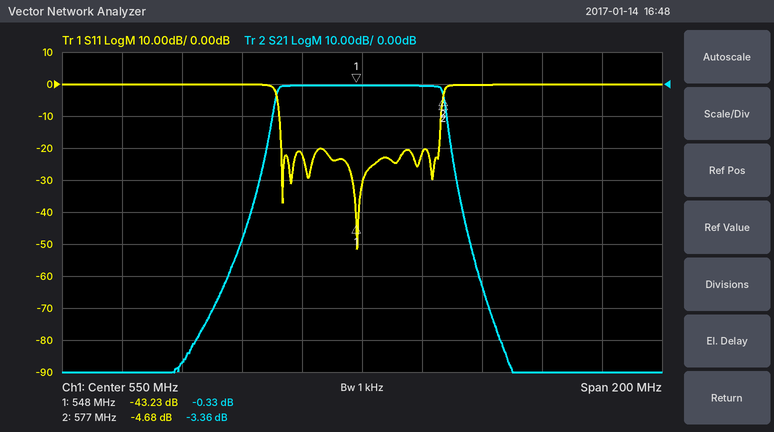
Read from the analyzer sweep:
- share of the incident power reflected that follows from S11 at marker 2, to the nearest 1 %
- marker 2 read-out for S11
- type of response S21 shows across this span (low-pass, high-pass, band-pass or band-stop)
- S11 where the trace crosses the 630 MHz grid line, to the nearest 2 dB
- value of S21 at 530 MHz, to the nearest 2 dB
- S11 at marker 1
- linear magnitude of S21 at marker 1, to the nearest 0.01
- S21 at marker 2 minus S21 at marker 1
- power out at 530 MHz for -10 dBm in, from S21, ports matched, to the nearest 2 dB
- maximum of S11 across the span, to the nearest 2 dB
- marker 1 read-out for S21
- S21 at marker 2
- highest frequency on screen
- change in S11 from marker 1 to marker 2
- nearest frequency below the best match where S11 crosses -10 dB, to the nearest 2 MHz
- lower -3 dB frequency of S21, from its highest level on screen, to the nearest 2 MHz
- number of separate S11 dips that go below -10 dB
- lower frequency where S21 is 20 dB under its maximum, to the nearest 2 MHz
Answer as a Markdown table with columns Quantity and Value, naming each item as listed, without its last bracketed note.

| Quantity | Value |
|---|---|
| share of the incident power reflected that follows from S11 at marker 2, to the nearest 1 % | 34 % |
| marker 2 read-out for S11 | -4.68 dB |
| type of response S21 shows across this span | band-pass |
| S11 where the trace crosses the 630 MHz grid line, to the nearest 2 dB | 0 dB |
| value of S21 at 530 MHz, to the nearest 2 dB | 0 dB |
| S11 at marker 1 | -43.23 dB |
| linear magnitude of S21 at marker 1, to the nearest 0.01 | 0.96 |
| S21 at marker 2 minus S21 at marker 1 | -3.03 dB |
| power out at 530 MHz for -10 dBm in, from S21, ports matched, to the nearest 2 dB | -10 dBm |
| maximum of S11 across the span, to the nearest 2 dB | 0 dB |
| marker 1 read-out for S21 | -0.33 dB |
| S21 at marker 2 | -3.36 dB |
| highest frequency on screen | 650 MHz |
| change in S11 from marker 1 to marker 2 | 38.55 dB |
| nearest frequency below the best match where S11 crosses -10 dB, to the nearest 2 MHz | 522 MHz |
| lower -3 dB frequency of S21, from its highest level on screen, to the nearest 2 MHz | 522 MHz |
| number of separate S11 dips that go below -10 dB | 6 |
| lower frequency where S21 is 20 dB under its maximum, to the nearest 2 MHz | 518 MHz |
